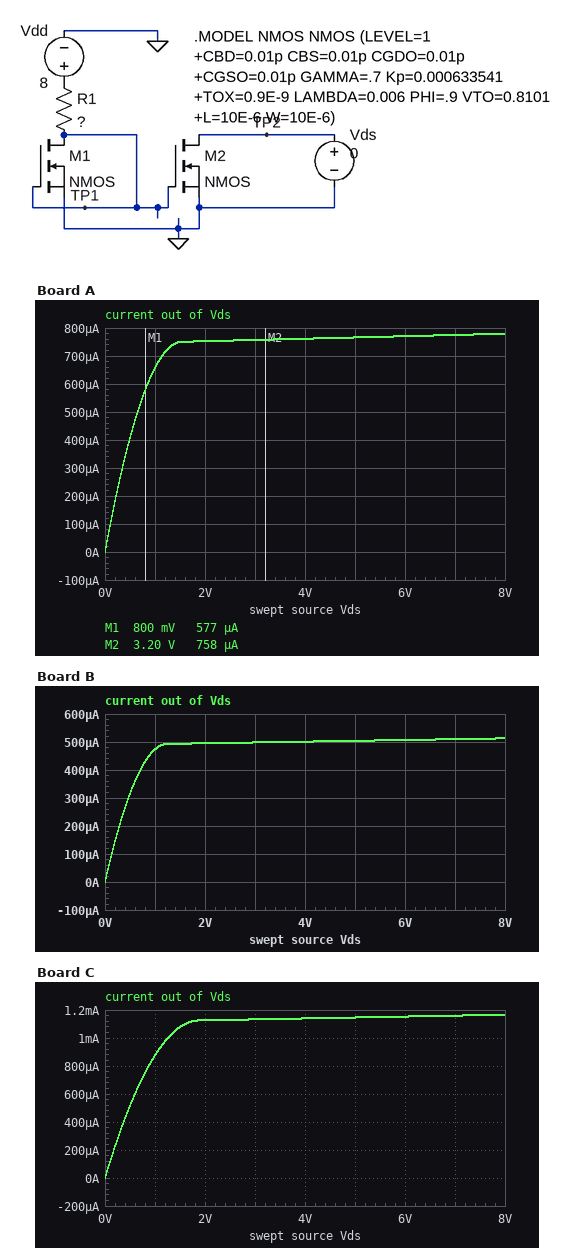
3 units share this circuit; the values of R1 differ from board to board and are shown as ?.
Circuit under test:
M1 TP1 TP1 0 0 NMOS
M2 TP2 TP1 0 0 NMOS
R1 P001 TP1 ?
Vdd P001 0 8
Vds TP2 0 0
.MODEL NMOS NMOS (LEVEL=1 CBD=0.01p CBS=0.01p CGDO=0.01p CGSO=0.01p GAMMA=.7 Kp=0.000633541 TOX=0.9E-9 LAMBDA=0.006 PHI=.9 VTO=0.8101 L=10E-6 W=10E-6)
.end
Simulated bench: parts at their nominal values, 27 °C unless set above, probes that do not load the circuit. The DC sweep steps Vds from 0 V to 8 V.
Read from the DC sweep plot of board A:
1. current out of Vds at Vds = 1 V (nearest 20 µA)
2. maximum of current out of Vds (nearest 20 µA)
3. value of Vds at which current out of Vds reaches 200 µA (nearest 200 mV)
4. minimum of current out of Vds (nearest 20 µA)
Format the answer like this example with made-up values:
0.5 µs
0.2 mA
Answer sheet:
660 µA
780 µA
200 mV
0 A
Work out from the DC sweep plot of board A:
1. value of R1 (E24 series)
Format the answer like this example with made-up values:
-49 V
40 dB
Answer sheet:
7.5 kΩ
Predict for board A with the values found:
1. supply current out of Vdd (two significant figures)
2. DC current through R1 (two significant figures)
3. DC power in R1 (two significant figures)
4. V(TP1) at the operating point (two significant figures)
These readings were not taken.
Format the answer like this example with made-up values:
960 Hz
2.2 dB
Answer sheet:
750 µA
750 µA
4.3 mW
2.3 V
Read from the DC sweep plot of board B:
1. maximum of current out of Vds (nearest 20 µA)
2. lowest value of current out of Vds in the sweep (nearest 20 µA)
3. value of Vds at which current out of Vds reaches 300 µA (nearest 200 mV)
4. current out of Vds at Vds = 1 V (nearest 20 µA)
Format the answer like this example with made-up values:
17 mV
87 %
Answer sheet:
520 µA
0 A
400 mV
480 µA
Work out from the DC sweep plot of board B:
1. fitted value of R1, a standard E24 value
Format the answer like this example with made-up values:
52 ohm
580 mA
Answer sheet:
12 kΩ
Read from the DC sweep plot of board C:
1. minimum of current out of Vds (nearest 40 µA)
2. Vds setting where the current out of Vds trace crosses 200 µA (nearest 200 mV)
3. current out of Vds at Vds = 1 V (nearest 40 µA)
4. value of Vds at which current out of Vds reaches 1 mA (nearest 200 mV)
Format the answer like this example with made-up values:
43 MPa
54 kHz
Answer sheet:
0 A
200 mV
880 µA
1.2 V
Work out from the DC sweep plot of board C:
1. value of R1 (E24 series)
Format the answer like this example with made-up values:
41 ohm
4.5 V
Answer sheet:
4.7 kΩ
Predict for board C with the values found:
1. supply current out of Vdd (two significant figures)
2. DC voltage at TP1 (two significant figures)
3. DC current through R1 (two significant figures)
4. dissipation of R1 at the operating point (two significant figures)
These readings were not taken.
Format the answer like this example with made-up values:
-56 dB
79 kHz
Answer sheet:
1.1 mA
2.7 V
1.1 mA
6.0 mW
